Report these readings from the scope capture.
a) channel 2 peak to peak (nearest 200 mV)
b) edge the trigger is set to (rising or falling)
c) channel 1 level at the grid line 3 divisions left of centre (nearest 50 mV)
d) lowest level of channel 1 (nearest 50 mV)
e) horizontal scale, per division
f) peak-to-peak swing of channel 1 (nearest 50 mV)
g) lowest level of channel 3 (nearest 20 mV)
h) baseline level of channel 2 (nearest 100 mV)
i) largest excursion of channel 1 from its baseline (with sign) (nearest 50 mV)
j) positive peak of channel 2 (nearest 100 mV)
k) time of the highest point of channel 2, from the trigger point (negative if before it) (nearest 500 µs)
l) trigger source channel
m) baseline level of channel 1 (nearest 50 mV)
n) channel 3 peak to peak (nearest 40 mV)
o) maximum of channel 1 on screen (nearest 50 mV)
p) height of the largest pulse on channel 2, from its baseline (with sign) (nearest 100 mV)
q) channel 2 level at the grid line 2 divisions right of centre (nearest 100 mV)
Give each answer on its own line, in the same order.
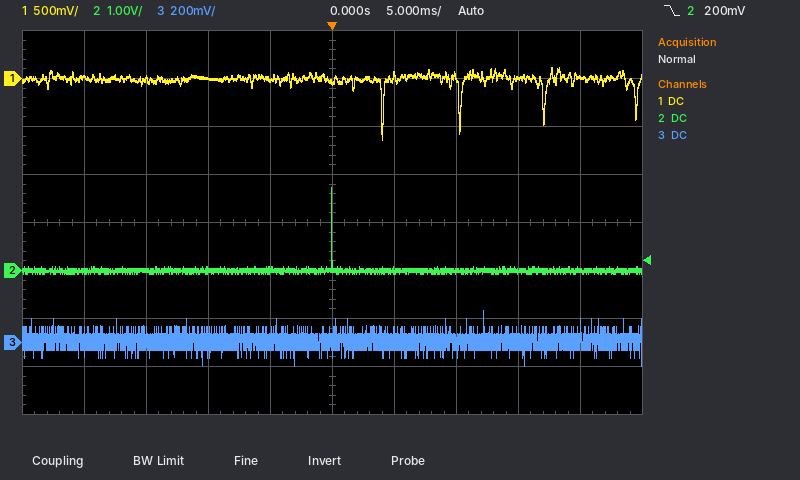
1.8 V
falling
0 mV
-650 mV
5 ms
750 mV
-100 mV
0.0 V
-650 mV
1.7 V
0.0 ms
channel 2
0 mV
240 mV
100 mV
+1.7 V
0.0 V
